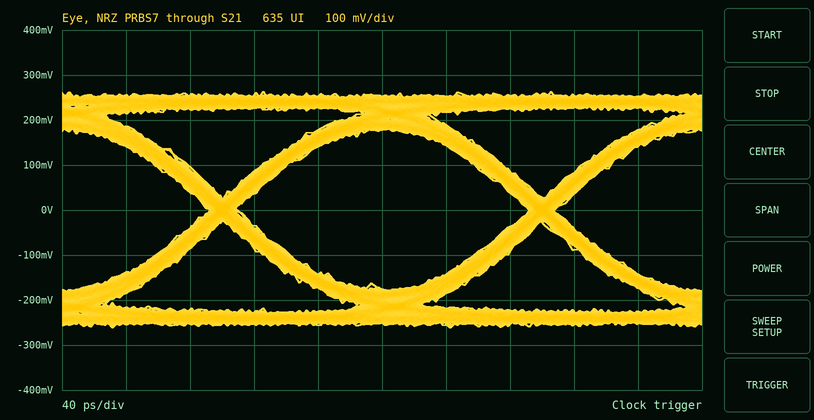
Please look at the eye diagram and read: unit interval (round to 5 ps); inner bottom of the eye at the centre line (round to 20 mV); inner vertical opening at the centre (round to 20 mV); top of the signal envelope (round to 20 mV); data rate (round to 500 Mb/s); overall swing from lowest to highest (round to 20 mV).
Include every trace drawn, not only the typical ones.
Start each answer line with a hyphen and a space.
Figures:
- 200 ps
- -180 mV
- 360 mV
- 260 mV
- 5.0 Gb/s
- 520 mV
